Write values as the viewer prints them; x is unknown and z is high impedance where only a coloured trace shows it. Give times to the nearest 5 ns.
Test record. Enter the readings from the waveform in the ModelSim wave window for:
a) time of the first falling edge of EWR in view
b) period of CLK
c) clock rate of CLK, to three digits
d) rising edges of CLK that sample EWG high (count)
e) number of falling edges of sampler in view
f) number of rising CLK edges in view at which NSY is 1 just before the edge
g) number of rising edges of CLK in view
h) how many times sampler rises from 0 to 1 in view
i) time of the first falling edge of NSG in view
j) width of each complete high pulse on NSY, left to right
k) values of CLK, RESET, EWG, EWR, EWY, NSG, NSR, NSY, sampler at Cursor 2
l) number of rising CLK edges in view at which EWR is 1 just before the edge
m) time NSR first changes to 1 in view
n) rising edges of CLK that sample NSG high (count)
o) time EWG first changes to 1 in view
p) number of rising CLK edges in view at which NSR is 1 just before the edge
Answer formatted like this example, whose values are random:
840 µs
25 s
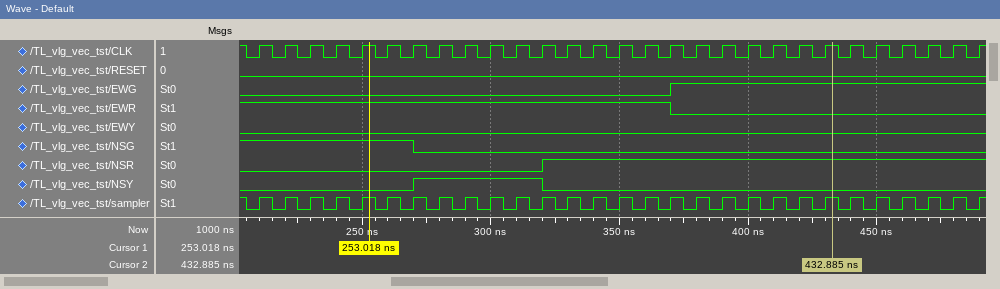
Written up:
370 ns
10 ns
100 MHz
12
29
5
29
29
270 ns
50 ns
CLK=1, RESET=0, EWG=1, EWR=0, EWY=0, NSG=0, NSR=1, NSY=0, sampler=1
17
320 ns
7
370 ns
17
